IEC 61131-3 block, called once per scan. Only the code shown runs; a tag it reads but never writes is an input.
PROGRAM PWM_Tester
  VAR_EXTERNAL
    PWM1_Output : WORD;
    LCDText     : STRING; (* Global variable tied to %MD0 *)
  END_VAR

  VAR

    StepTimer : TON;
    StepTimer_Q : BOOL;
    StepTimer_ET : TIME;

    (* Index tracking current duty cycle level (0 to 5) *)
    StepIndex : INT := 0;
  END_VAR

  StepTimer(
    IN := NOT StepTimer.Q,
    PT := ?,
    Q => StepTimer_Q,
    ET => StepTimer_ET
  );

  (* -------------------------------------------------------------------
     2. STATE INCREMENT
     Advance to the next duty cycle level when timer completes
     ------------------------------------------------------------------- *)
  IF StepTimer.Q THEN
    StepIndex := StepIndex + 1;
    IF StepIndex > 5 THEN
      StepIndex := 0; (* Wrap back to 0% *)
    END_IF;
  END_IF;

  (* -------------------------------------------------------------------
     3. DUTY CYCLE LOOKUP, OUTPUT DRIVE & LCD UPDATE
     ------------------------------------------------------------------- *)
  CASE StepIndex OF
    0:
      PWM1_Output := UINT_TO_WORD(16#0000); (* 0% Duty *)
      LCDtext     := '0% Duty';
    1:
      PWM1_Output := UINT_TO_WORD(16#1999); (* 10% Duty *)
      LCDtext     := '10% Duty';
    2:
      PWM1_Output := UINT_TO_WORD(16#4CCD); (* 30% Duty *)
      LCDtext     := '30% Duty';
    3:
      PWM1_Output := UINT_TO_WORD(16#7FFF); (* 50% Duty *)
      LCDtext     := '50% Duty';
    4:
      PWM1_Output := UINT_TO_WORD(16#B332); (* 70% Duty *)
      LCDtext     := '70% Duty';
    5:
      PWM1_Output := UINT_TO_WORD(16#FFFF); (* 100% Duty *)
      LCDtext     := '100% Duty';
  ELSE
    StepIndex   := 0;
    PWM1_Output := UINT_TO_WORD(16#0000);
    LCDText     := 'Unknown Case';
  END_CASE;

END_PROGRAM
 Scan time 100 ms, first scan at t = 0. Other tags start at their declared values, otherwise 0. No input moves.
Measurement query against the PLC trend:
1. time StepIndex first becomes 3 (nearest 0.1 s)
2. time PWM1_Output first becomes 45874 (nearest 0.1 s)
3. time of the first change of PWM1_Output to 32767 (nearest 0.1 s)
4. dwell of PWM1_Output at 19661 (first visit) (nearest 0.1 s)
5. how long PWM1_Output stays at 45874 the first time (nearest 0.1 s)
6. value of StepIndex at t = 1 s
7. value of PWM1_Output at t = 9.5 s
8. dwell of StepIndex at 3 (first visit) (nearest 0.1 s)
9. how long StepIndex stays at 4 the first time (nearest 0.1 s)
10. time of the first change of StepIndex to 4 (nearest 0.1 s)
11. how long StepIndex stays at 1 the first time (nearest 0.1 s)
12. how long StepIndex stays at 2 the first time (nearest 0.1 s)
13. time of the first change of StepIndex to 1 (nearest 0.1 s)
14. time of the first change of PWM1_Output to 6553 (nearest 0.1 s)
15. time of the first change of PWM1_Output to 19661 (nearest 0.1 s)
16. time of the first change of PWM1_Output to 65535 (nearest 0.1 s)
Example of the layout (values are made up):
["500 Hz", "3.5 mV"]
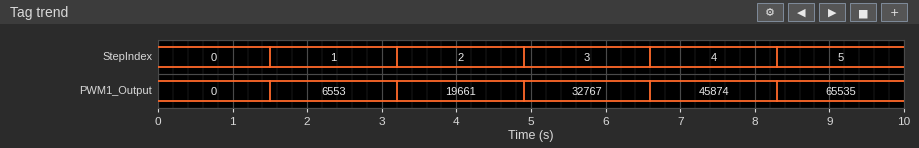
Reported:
["4.9 s", "6.6 s", "4.9 s", "1.7 s", "1.7 s", "0", "65535", "1.7 s", "1.7 s", "6.6 s", "1.7 s", "1.7 s", "1.5 s", "1.5 s", "3.2 s", "8.3 s"]
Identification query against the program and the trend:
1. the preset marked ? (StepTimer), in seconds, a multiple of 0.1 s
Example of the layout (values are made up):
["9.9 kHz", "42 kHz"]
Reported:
["1.5 s"]
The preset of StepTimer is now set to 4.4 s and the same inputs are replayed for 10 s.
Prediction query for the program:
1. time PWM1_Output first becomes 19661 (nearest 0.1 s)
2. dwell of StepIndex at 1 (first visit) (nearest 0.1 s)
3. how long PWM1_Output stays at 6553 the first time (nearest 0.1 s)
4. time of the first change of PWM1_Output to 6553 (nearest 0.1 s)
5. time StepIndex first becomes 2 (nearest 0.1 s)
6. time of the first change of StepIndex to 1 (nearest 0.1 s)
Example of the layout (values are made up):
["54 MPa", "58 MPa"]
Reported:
["9.0 s", "4.6 s", "4.6 s", "4.4 s", "9.0 s", "4.4 s"]
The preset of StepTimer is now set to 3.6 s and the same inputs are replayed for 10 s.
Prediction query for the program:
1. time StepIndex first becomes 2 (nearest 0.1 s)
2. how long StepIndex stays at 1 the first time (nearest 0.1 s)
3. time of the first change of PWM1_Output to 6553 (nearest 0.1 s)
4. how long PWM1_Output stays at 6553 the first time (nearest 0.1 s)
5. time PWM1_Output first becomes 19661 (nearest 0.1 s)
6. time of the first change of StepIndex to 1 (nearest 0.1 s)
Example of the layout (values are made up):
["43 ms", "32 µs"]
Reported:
["7.4 s", "3.8 s", "3.6 s", "3.8 s", "7.4 s", "3.6 s"]
